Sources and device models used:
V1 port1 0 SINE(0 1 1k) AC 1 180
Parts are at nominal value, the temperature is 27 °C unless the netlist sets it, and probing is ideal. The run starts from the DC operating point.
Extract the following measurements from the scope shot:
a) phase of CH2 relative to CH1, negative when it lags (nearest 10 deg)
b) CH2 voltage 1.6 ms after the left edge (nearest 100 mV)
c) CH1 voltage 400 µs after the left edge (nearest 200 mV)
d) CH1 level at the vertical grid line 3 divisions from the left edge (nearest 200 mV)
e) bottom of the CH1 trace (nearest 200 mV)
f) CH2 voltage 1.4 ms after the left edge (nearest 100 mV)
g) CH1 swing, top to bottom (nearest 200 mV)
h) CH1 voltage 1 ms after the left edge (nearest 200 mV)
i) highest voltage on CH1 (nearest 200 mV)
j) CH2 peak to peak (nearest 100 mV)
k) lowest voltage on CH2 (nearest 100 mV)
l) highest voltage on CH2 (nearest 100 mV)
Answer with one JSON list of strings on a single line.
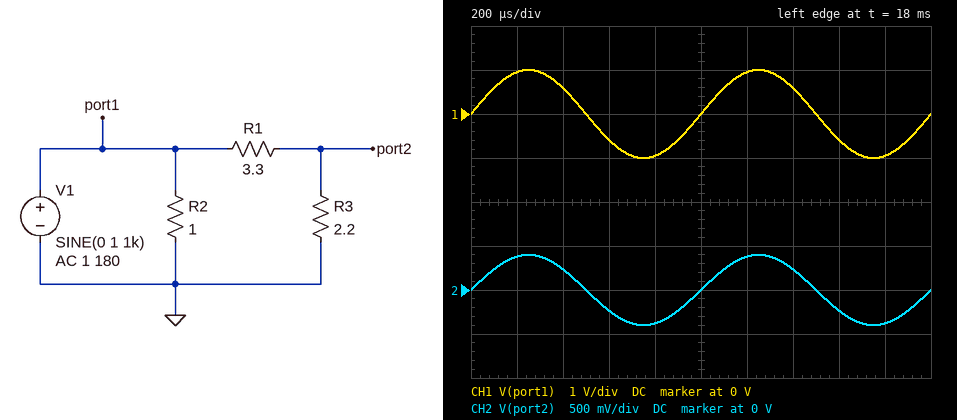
["0 deg", "-200 mV", "600 mV", "-600 mV", "-1.0 V", "200 mV", "2.0 V", "0 V", "1.0 V", "800 mV", "-400 mV", "400 mV"]
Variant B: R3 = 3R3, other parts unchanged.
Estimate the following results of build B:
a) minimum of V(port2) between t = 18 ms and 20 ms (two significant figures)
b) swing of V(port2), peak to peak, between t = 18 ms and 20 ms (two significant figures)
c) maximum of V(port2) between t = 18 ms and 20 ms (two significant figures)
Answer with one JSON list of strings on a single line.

["-500 mV", "1.0 V", "500 mV"]
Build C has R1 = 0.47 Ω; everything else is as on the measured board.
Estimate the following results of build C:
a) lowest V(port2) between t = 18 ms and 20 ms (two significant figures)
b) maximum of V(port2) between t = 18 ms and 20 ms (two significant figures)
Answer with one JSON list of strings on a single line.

["-820 mV", "820 mV"]
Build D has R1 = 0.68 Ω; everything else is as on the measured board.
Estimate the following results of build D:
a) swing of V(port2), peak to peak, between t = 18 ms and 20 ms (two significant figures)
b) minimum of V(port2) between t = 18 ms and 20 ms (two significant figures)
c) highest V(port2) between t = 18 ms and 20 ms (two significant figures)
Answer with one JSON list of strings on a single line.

["1.5 V", "-760 mV", "760 mV"]
